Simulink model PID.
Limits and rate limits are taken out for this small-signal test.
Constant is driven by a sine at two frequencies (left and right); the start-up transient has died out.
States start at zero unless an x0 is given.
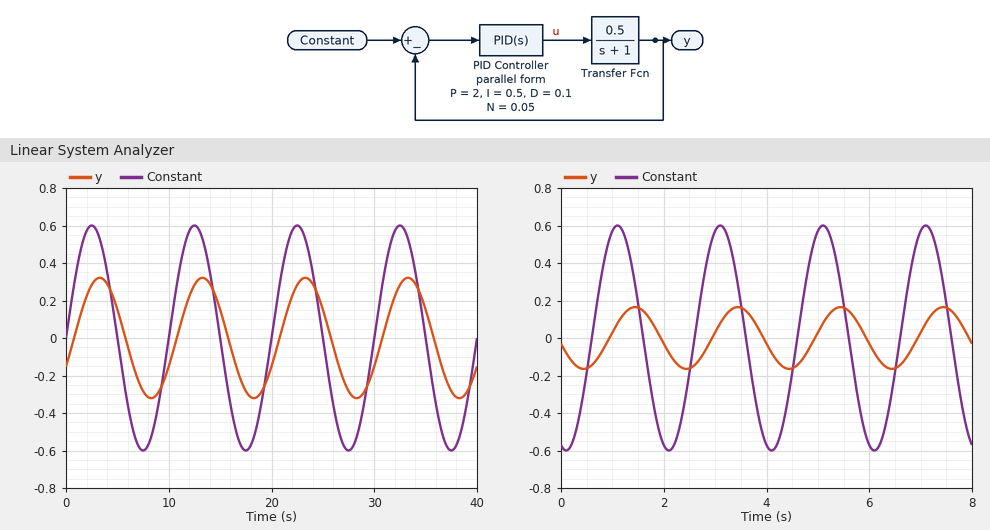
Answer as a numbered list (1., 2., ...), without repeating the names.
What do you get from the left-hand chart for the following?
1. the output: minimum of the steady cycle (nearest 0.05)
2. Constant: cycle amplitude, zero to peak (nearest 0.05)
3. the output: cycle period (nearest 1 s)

1. -0.30
2. 0.60
3. 10 s
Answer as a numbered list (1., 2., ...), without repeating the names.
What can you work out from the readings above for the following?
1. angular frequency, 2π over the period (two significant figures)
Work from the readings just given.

1. 0.63 rad/s
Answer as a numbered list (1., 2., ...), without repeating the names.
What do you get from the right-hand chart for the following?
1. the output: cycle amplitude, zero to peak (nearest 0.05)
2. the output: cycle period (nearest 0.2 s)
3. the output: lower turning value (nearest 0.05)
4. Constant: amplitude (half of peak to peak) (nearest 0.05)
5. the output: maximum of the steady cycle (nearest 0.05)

1. 0.15
2. 2.0 s
3. -0.15
4. 0.60
5. 0.15
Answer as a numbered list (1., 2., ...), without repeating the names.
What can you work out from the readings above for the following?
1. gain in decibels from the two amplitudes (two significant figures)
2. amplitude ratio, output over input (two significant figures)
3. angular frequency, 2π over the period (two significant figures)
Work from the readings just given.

1. -12 dB
2. 0.25
3. 3.1 rad/s
